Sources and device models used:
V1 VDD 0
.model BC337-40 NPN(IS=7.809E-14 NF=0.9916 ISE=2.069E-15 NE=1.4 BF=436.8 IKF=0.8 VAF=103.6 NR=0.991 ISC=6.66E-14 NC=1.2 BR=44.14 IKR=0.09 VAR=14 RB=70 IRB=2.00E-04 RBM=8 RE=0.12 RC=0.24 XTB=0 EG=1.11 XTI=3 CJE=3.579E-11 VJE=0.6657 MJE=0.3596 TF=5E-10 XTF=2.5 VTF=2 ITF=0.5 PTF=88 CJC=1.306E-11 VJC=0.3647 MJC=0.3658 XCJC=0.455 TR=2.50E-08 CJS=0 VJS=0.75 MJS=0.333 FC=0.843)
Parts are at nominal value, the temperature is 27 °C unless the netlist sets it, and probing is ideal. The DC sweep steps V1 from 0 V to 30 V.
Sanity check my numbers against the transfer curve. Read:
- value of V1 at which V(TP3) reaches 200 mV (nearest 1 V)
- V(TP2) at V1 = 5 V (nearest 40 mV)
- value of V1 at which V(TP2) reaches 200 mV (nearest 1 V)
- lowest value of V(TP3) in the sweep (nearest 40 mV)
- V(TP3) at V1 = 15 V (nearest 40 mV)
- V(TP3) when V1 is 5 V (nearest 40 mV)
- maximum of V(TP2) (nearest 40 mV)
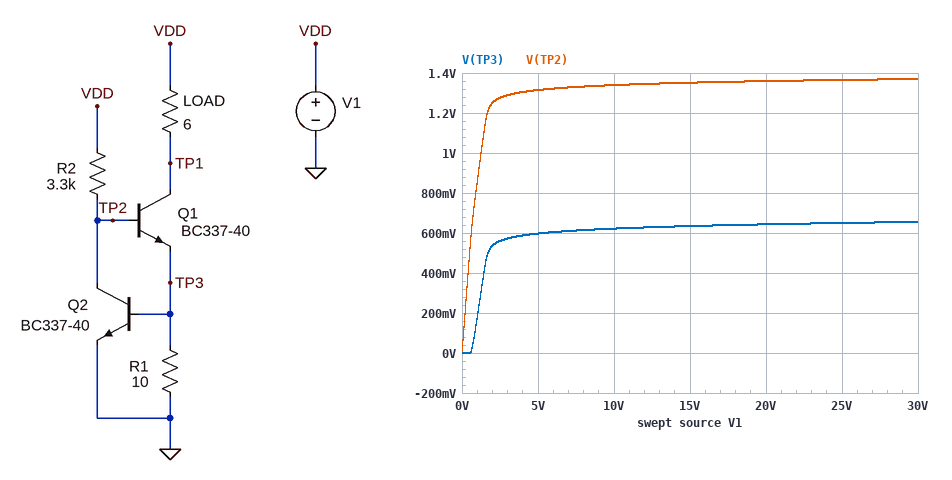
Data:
1 V
1.32 V
0 V
0 V
640 mV
600 mV
1.36 V
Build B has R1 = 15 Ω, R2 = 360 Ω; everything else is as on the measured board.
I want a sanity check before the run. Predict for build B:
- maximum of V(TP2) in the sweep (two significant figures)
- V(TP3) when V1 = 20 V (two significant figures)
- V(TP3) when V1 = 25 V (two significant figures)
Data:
1.4 V
710 mV
720 mV
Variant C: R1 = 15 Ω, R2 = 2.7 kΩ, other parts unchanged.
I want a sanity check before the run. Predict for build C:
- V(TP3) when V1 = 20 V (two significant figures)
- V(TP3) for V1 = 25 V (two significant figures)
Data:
650 mV
660 mV
